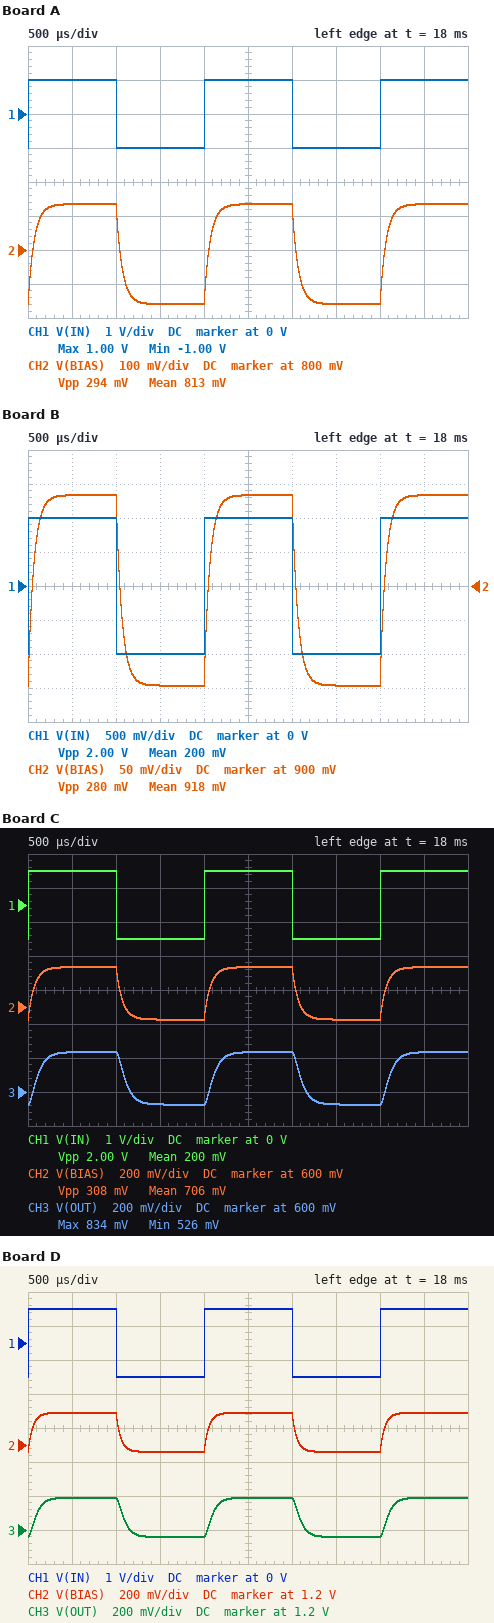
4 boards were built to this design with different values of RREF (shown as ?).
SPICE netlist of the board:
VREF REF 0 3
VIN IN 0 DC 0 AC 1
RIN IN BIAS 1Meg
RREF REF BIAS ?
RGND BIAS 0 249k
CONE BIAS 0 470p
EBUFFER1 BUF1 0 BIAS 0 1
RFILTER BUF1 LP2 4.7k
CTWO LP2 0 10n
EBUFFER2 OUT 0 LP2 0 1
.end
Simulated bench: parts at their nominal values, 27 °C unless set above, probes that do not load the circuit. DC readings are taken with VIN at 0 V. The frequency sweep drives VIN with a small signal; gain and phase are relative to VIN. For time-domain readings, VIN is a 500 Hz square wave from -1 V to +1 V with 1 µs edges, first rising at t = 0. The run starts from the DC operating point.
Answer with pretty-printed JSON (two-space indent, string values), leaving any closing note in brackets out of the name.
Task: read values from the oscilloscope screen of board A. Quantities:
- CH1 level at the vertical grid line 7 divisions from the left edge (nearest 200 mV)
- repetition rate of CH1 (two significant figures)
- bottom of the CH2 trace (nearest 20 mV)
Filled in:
{
  "CH1 level at the vertical grid line 7 divisions from the left edge": "-1.0 V",
  "repetition rate of CH1": "500 Hz",
  "bottom of the CH2 trace": "640 mV"
}
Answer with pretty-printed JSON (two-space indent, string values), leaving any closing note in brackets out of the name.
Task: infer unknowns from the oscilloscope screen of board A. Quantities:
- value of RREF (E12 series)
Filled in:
{
  "value of RREF": "560 kΩ"
}
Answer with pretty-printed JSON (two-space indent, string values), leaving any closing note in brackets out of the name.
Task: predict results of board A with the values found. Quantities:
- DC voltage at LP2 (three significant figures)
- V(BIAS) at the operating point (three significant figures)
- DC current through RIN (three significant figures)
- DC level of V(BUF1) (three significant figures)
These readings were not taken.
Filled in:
{
  "DC voltage at LP2": "788 mV",
  "V(BIAS) at the operating point": "788 mV",
  "DC current through RIN": "788 nA",
  "DC level of V(BUF1)": "788 mV"
}
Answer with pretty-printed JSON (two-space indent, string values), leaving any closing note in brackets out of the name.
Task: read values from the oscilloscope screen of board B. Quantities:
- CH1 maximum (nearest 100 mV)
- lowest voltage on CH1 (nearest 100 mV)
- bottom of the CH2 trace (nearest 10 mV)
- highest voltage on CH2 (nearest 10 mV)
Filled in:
{
  "CH1 maximum": "1.0 V",
  "lowest voltage on CH1": "-1.0 V",
  "bottom of the CH2 trace": "750 mV",
  "highest voltage on CH2": "1.03 V"
}
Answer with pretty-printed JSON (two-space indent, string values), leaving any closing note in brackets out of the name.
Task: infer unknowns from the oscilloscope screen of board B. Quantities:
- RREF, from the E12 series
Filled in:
{
  "RREF, from the E12 series": "470 kΩ"
}
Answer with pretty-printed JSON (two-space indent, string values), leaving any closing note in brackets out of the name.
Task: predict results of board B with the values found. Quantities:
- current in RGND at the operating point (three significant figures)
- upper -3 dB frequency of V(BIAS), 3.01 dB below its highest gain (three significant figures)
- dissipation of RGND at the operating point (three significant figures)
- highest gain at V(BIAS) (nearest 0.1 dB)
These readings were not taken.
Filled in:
{
  "current in RGND at the operating point": "3.59 µA",
  "upper -3 dB frequency of V(BIAS), 3.01 dB below its highest gain": "2.42 kHz",
  "dissipation of RGND at the operating point": "3.21 µW",
  "highest gain at V(BIAS)": "-17.1 dB"
}
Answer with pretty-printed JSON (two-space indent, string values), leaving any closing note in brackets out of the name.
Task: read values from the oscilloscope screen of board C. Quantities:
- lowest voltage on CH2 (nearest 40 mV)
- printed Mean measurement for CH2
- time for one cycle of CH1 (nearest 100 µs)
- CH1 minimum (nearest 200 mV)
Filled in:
{
  "lowest voltage on CH2": "520 mV",
  "printed Mean measurement for CH2": "706 mV",
  "time for one cycle of CH1": "2.0 ms",
  "CH1 minimum": "-1.0 V"
}
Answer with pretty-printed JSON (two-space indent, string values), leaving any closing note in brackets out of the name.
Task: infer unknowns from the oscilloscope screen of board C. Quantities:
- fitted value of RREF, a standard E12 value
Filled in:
{
  "fitted value of RREF, a standard E12 value": "680 kΩ"
}
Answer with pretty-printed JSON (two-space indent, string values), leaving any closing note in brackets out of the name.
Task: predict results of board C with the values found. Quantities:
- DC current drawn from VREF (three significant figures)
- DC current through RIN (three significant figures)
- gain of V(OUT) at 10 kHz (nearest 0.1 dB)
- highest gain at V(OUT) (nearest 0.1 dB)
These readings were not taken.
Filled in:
{
  "DC current drawn from VREF": "3.41 µA",
  "DC current through RIN": "680 nA",
  "gain of V(OUT) at 10 kHz": "-39.5 dB",
  "highest gain at V(OUT)": "-16.2 dB"
}
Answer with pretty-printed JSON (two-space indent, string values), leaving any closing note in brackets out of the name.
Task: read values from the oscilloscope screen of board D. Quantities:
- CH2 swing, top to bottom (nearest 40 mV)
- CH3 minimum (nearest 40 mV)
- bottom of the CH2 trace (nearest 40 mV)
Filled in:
{
  "CH2 swing, top to bottom": "240 mV",
  "CH3 minimum": "1.16 V",
  "bottom of the CH2 trace": "1.16 V"
}
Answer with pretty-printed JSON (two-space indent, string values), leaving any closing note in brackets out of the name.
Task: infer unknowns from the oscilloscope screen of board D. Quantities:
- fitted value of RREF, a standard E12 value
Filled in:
{
  "fitted value of RREF, a standard E12 value": "270 kΩ"
}
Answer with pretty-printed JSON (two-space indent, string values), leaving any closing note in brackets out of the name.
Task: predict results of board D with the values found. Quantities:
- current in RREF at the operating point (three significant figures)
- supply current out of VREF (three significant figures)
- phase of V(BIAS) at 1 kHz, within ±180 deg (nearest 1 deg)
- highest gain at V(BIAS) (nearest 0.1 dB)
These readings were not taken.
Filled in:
{
  "current in RREF at the operating point": "6.39 µA",
  "supply current out of VREF": "6.39 µA",
  "phase of V(BIAS) at 1 kHz, within ±180 deg": "-19 deg",
  "highest gain at V(BIAS)": "-18.8 dB"
}
